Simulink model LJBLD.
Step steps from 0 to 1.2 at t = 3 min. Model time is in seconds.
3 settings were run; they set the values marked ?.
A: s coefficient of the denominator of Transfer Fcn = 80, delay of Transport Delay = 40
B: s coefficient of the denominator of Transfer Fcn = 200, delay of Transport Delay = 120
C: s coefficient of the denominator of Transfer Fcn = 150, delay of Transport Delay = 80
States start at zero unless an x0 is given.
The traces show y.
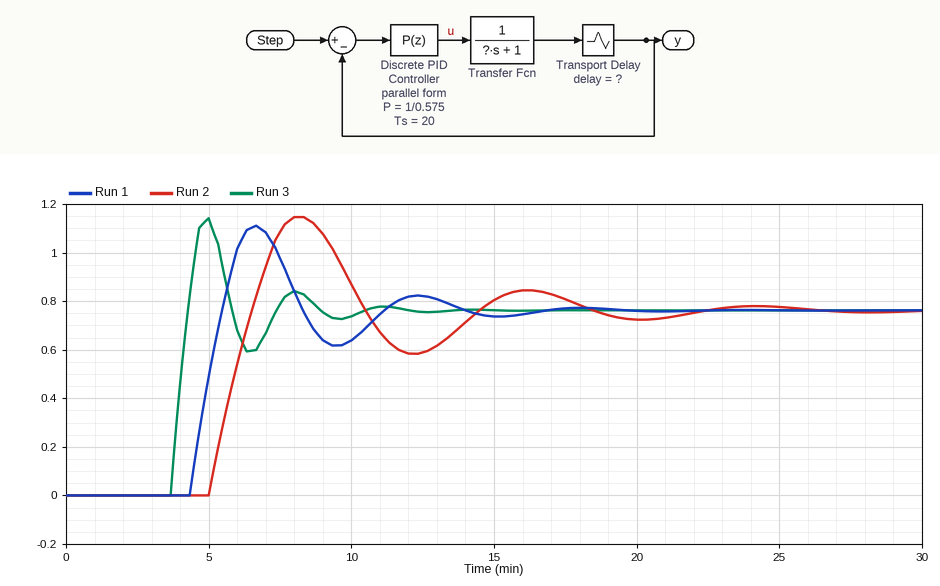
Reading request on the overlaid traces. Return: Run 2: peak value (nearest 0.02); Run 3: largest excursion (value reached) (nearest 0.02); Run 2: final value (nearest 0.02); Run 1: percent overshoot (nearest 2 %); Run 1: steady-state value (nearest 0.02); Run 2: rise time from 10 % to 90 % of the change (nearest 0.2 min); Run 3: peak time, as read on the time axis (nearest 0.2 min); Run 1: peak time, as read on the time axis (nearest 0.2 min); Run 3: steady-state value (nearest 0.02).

1.14
1.14
0.76
46 %
0.76
1.2 min
5.0 min
6.6 min
0.76
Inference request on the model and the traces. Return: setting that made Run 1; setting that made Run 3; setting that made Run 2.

C
A
B
